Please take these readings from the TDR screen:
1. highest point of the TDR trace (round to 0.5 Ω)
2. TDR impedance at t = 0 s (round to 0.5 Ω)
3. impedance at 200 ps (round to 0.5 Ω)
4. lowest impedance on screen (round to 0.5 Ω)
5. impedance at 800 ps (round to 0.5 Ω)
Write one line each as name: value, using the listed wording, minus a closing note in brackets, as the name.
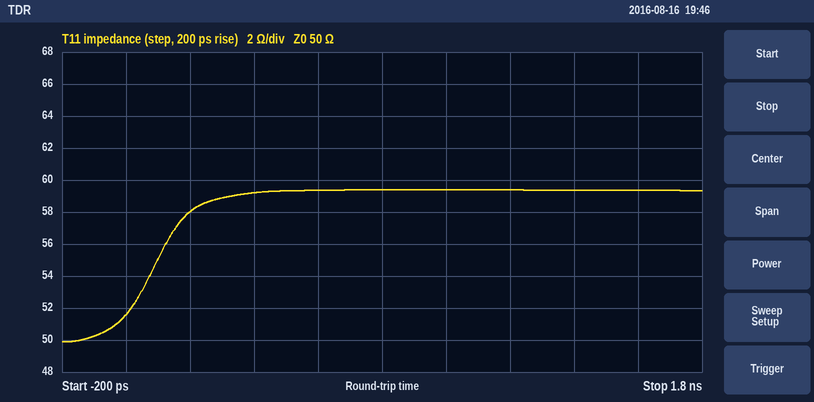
highest point of the TDR trace: 59.5 Ω
TDR impedance at t = 0 s: 51.5 Ω
impedance at 200 ps: 58.0 Ω
lowest impedance on screen: 50.0 Ω
impedance at 800 ps: 59.5 Ω
